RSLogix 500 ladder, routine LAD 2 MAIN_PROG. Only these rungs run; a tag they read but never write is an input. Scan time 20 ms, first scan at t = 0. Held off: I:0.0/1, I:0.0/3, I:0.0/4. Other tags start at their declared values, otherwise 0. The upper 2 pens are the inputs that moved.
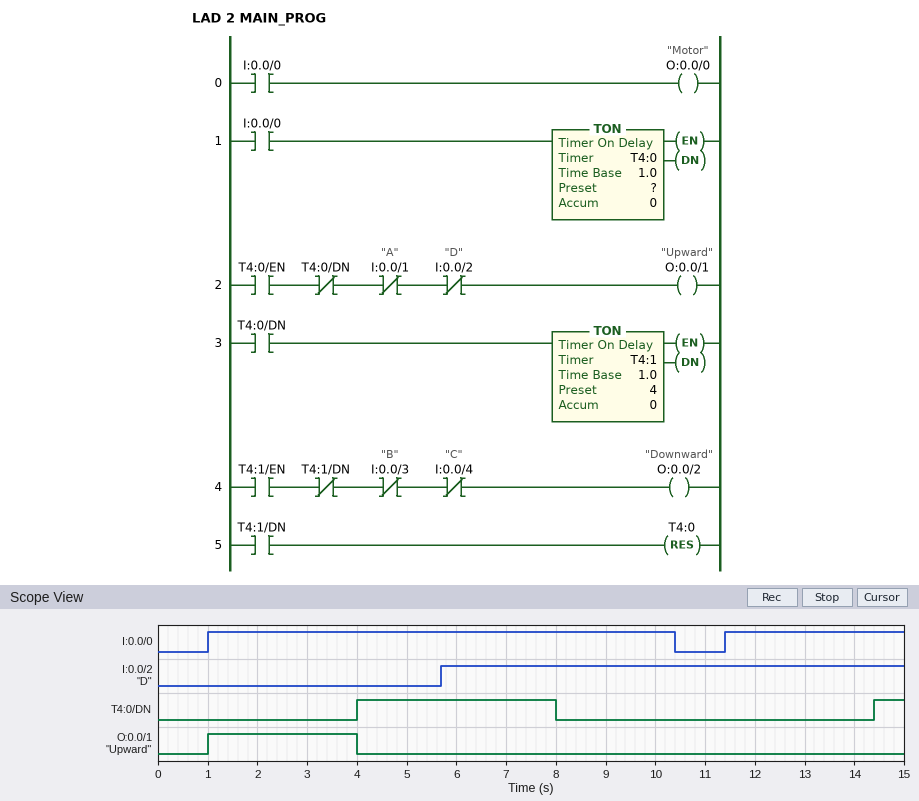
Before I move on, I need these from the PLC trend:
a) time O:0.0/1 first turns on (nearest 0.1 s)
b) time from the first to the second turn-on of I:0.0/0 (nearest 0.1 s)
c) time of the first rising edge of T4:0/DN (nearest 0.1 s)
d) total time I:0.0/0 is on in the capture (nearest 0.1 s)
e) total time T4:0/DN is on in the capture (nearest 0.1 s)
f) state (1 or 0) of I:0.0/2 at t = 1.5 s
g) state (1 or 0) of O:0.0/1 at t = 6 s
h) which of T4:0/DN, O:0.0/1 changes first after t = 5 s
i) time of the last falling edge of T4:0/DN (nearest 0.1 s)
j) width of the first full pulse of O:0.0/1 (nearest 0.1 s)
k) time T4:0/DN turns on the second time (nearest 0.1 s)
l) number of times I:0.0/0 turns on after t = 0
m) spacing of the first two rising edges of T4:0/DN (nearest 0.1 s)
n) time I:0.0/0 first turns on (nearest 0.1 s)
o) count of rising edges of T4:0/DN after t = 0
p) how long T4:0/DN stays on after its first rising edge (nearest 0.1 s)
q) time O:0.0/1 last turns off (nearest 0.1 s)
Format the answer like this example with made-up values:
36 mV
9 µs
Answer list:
1.0 s
10.4 s
4.0 s
13.0 s
4.6 s
0
0
T4:0/DN
8.0 s
3.0 s
14.4 s
2
10.4 s
1.0 s
2
4.0 s
4.0 s
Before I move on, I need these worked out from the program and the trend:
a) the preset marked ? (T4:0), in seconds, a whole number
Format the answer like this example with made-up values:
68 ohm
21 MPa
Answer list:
3 s
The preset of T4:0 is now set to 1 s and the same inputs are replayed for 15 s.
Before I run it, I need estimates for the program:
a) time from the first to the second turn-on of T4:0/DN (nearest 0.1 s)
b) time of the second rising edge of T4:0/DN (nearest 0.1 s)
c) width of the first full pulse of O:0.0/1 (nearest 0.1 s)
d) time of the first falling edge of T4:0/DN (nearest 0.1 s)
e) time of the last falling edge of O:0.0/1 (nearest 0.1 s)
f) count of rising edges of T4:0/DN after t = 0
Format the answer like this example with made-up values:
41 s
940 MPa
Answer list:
5.0 s
7.0 s
1.0 s
6.0 s
2.0 s
3
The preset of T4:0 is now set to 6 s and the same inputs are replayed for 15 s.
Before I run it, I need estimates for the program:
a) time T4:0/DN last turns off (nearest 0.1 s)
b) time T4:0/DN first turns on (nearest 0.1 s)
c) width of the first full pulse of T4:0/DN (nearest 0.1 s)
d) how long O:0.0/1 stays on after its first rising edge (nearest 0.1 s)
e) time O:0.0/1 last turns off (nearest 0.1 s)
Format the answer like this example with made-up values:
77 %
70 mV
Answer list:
10.4 s
7.0 s
3.4 s
4.7 s
5.7 s
